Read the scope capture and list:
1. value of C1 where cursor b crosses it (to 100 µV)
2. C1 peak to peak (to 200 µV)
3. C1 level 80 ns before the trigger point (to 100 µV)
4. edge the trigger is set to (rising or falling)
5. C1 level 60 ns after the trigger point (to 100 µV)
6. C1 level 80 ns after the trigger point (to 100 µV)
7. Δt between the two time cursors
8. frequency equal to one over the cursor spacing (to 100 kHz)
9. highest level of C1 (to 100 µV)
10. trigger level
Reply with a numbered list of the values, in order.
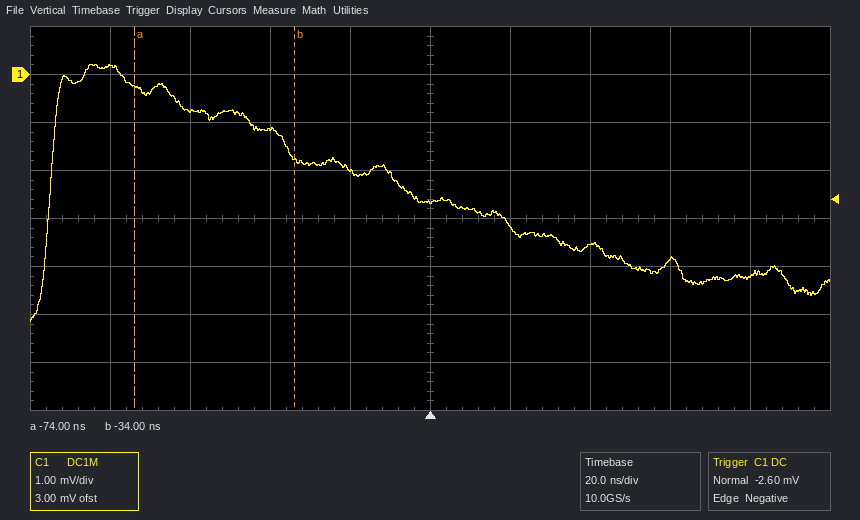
1. -1.8 mV
2. 5.4 mV
3. 200 µV
4. falling
5. -3.9 mV
6. -4.2 mV
7. 40 ns
8. 25.0 MHz
9. 200 µV
10. -2.60 mV
